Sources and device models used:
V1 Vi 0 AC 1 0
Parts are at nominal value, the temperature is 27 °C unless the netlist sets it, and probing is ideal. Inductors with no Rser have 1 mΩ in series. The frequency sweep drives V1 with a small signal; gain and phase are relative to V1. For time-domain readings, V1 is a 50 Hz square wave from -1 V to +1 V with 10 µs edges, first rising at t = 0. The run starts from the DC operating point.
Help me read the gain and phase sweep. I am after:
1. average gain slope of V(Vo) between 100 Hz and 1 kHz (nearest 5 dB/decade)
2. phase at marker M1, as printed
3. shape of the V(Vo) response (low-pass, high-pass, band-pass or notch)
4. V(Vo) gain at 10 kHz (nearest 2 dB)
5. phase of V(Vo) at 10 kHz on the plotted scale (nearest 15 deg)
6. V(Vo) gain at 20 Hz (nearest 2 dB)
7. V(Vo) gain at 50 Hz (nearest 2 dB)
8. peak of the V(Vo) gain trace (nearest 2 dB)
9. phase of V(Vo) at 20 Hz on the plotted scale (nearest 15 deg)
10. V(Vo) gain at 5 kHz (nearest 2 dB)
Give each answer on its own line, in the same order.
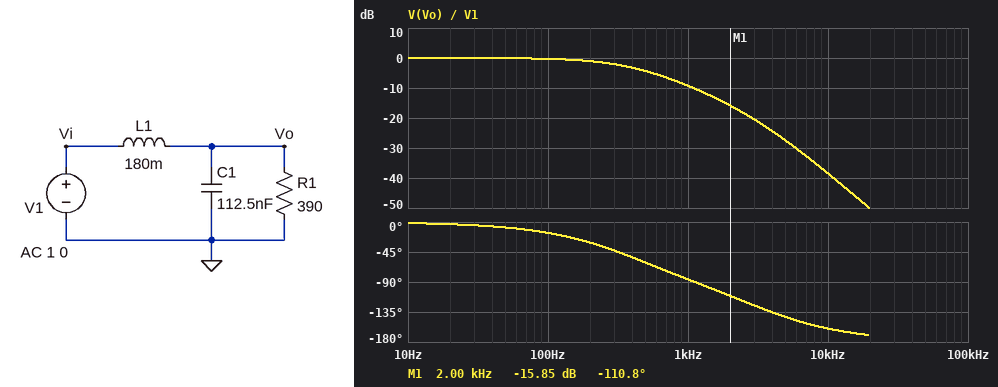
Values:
-10 dB/decade
-110.8 deg
low-pass
-38 dB
-165 deg
0 dB
0 dB
0 dB
0 deg
-28 dB
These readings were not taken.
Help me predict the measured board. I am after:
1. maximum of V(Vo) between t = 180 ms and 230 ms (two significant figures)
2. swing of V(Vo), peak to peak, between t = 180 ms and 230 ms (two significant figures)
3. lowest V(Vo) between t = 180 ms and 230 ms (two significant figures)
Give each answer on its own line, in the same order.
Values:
1.0 V
2.0 V
-1.0 V
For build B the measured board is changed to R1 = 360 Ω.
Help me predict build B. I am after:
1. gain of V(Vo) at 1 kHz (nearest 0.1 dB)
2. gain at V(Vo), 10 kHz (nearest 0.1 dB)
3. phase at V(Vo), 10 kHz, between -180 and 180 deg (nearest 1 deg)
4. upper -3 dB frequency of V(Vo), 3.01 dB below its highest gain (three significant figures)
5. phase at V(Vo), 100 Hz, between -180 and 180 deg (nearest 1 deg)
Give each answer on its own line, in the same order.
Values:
-10.0 dB
-38.6 dB
-158 deg
346 Hz
-18 deg
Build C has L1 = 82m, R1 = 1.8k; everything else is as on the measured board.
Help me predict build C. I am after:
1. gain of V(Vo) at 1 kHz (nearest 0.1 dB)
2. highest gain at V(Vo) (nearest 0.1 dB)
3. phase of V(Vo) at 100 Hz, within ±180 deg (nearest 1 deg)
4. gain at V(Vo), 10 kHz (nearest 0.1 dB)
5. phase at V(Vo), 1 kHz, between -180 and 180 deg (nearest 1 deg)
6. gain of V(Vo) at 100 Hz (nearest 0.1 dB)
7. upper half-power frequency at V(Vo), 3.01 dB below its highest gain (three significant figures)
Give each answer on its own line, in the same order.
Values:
3.1 dB
6.7 dB
-2 deg
-31.0 dB
-24 deg
0 dB
1.92 kHz
